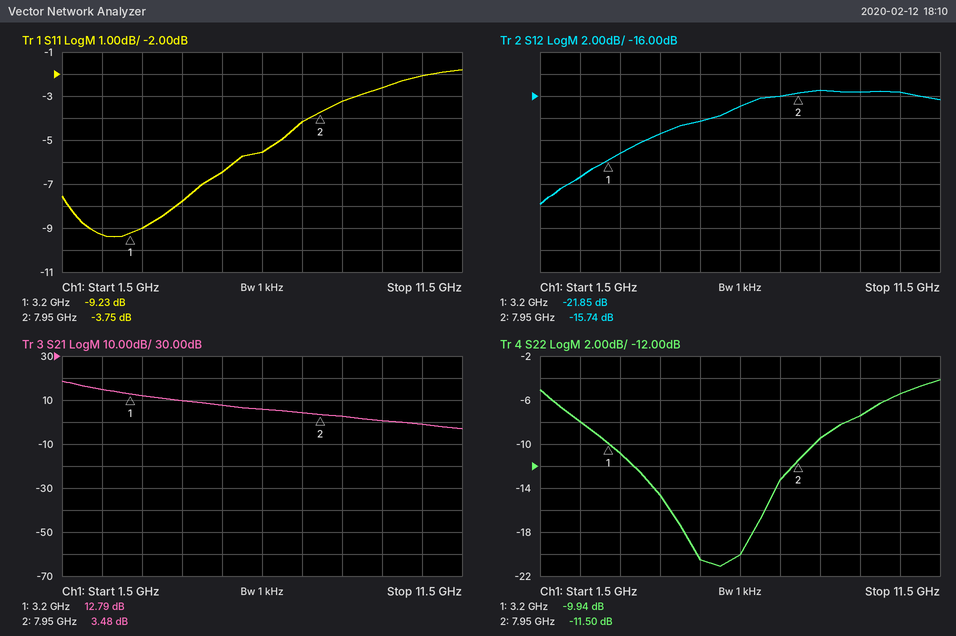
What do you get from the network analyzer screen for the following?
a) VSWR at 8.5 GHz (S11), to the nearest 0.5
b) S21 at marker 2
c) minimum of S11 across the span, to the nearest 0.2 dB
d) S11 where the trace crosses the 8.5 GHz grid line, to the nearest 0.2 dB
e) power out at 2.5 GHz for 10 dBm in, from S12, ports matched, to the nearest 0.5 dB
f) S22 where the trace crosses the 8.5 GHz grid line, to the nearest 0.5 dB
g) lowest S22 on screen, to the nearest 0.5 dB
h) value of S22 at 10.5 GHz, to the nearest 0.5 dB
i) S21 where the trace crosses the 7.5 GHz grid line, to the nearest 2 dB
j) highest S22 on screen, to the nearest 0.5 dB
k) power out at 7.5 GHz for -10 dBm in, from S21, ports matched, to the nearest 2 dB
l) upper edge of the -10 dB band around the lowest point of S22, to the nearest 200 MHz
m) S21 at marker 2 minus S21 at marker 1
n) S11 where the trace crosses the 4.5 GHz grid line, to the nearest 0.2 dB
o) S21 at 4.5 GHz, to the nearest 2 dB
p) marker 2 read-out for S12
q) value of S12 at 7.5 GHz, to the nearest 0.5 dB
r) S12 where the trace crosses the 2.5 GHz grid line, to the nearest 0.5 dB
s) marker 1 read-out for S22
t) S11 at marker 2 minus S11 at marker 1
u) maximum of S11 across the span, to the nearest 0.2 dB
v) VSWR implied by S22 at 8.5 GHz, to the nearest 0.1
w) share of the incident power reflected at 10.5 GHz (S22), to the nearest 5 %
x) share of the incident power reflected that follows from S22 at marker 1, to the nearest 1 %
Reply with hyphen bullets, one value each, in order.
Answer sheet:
- 5.5
- 3.48 dB
- -9.4 dB
- -3.2 dB
- -13.5 dBm
- -9.5 dB
- -21.0 dB
- -5.5 dB
- 4 dB
- -4.0 dB
- -6 dBm
- 8.4 GHz
- -9.31 dB
- -7.8 dB
- 10 dB
- -15.74 dB
- -16.0 dB
- -23.5 dB
- -9.94 dB
- 5.48 dB
- -1.8 dB
- 2.0
- 30 %
- 10 %
